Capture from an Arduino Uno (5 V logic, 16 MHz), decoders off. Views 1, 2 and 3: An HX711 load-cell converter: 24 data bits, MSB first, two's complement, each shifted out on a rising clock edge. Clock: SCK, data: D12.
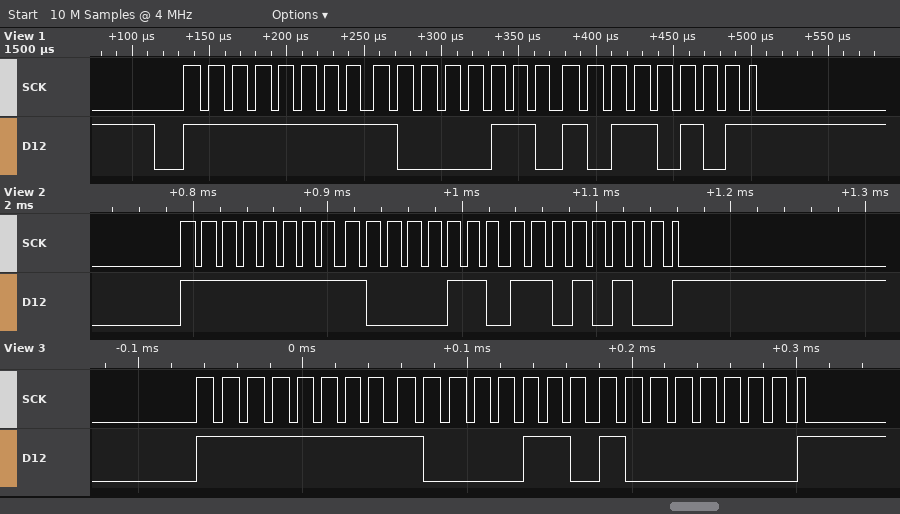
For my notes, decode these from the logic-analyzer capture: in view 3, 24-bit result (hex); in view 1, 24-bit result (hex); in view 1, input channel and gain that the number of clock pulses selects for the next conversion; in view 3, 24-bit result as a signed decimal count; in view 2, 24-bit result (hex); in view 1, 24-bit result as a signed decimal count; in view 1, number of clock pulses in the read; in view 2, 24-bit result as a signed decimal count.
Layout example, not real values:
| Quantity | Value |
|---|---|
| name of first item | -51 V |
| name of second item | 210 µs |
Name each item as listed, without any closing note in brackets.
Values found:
| Quantity | Value |
|---|---|
| in view 3, 24-bit result | 0xFF8680 |
| in view 1, 24-bit result | 0xFF86B5 |
| in view 1, input channel and gain that the number of clock pulses selects for the next conversion | channel A, gain 128 |
| in view 3, 24-bit result as a signed decimal count | -31104 |
| in view 2, 24-bit result | 0xFF86D4 |
| in view 1, 24-bit result as a signed decimal count | -31051 |
| in view 1, number of clock pulses in the read | 25 |
| in view 2, 24-bit result as a signed decimal count | -31020 |
